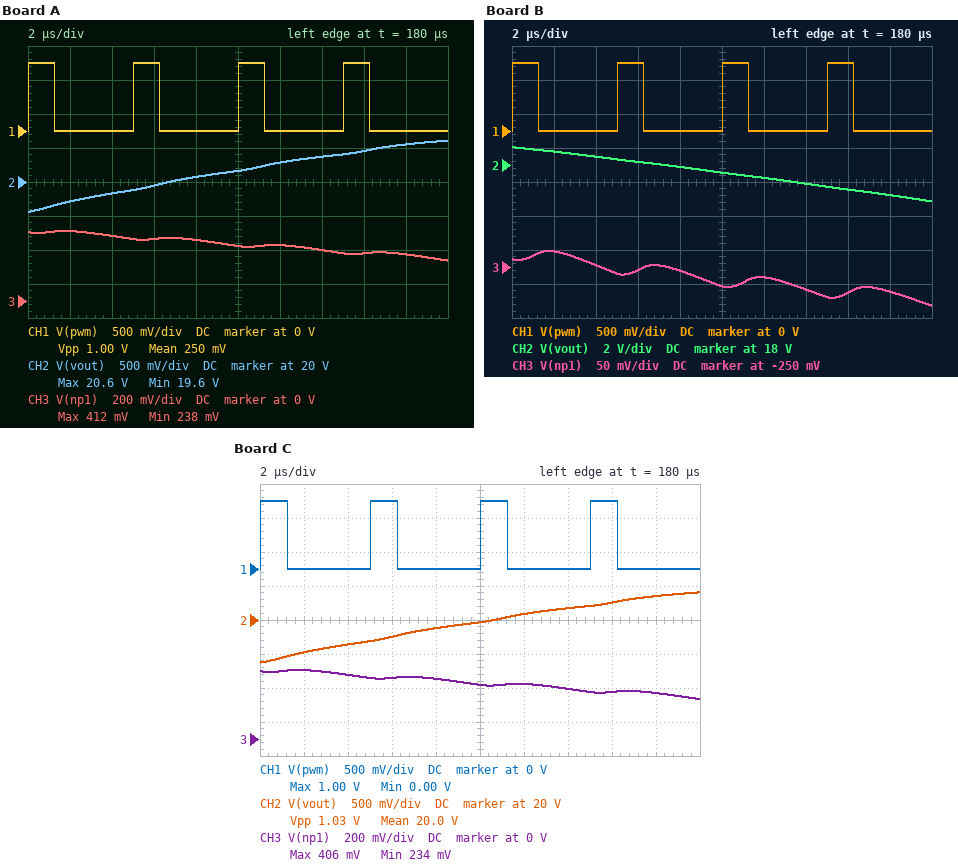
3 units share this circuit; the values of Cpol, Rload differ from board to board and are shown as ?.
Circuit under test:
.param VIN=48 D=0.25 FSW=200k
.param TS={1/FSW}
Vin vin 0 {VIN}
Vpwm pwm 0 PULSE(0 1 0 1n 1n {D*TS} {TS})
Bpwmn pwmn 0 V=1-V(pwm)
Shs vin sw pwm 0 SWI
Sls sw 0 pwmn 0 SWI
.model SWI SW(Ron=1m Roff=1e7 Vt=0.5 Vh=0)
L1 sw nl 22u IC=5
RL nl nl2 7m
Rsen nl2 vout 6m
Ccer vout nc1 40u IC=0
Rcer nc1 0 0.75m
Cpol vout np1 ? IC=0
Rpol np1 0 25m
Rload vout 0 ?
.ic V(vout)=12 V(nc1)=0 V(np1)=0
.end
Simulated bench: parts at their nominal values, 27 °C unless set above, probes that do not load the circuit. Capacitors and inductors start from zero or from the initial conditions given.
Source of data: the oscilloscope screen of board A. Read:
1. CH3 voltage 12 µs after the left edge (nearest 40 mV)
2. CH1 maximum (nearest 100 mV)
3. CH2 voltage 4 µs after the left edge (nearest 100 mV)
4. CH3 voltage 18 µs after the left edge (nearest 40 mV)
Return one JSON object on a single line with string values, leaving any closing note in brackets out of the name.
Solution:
{"CH3 voltage 12 µs after the left edge": "320 mV", "CH1 maximum": "1.0 V", "CH2 voltage 4 µs after the left edge": "19.8 V", "CH3 voltage 18 µs after the left edge": "280 mV"}
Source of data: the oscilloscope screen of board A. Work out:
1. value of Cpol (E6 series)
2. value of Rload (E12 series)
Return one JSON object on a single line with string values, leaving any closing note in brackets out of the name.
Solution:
{"value of Cpol": "220 µF", "value of Rload": "3.9 Ω"}
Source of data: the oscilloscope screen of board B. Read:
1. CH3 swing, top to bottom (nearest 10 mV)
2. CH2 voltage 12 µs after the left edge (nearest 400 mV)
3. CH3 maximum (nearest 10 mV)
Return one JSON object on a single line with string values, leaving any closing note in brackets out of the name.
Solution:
{"CH3 swing, top to bottom": "80 mV", "CH2 voltage 12 µs after the left edge": "17.2 V", "CH3 maximum": "-230 mV"}
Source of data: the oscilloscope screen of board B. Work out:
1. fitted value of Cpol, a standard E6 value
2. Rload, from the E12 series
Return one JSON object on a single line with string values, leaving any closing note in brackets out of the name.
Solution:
{"fitted value of Cpol, a standard E6 value": "68 µF", "Rload, from the E12 series": "5.6 Ω"}
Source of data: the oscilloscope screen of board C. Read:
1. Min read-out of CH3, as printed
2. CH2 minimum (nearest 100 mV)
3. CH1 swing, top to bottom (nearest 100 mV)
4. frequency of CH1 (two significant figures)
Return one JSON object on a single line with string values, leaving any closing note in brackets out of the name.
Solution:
{"Min read-out of CH3, as printed": "234 mV", "CH2 minimum": "19.4 V", "CH1 swing, top to bottom": "1.0 V", "frequency of CH1": "200 kHz"}
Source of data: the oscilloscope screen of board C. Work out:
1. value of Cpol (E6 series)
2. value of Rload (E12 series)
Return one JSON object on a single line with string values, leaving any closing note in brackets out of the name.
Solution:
{"value of Cpol": "220 µF", "value of Rload": "3.3 Ω"}
